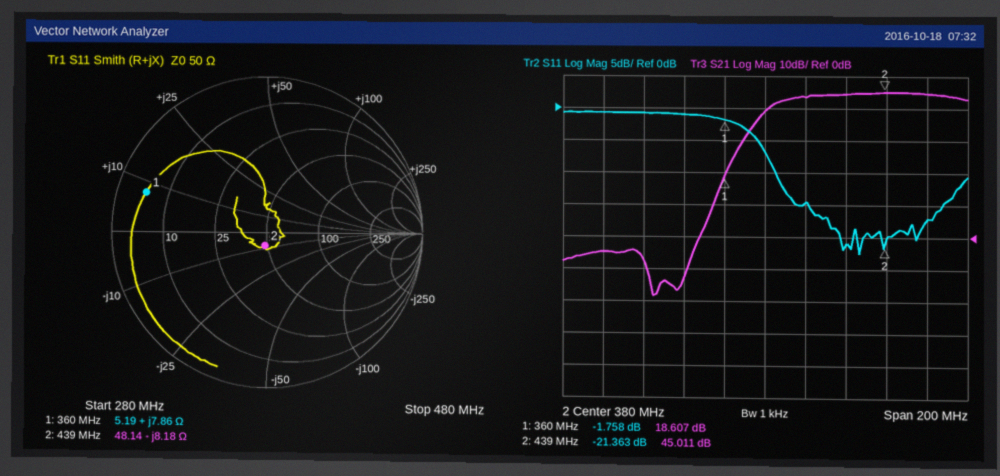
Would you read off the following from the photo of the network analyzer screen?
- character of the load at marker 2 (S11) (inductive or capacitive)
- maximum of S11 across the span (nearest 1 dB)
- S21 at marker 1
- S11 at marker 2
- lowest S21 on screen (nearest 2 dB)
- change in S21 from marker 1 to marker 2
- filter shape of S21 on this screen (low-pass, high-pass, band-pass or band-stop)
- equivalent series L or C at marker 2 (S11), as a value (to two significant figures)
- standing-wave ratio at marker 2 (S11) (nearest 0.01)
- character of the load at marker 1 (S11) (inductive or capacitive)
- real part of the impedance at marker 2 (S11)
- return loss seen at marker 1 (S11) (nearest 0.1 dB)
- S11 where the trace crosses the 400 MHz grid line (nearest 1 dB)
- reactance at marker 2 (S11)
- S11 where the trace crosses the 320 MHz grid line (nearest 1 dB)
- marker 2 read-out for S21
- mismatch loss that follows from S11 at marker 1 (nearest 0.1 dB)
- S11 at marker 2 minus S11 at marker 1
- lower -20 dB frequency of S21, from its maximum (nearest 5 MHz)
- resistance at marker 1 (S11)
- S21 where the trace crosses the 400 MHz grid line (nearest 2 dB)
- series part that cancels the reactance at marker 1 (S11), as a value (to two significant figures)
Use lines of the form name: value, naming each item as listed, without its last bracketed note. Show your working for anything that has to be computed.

character of the load at marker 2 (S11): capacitive
maximum of S11 across the span: -1 dB
S21 at marker 1: 18.607 dB
S11 at marker 2: -21.363 dB
lowest S21 on screen: -18 dB
change in S21 from marker 1 to marker 2: 45.011 − (18.607) = 26.404 dB
filter shape of S21 on this screen: high-pass
equivalent series L or C at marker 2 (S11), as a value: C = 1/(2π × 439 MHz × 8.18 Ω) ≈ 44 pF
standing-wave ratio at marker 2 (S11): 1.19
character of the load at marker 1 (S11): inductive
real part of the impedance at marker 2: 48.14 Ω
return loss seen at marker 1 (S11): 1.8 dB
S11 where the trace crosses the 400 MHz grid line: -15 dB
reactance at marker 2: -8.18 Ω
S11 where the trace crosses the 320 MHz grid line: -1 dB
marker 2 read-out for S21: 45.011 dB
mismatch loss that follows from S11 at marker 1: −10 log10(1 − 10^(-1.758/10)) ≈ 4.8 dB
S11 at marker 2 minus S11 at marker 1: -21.363 − (-1.758) = -19.605 dB
lower -20 dB frequency of S21, from its maximum: 365 MHz
resistance at marker 1: 5.19 Ω
S21 where the trace crosses the 400 MHz grid line: 44 dB
series part that cancels the reactance at marker 1 (S11), as a value: C = 1/(2π × 360 MHz × 7.86 Ω) ≈ 56 pF
